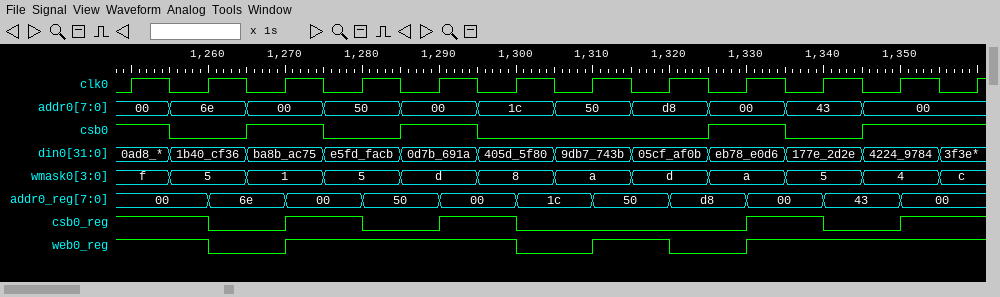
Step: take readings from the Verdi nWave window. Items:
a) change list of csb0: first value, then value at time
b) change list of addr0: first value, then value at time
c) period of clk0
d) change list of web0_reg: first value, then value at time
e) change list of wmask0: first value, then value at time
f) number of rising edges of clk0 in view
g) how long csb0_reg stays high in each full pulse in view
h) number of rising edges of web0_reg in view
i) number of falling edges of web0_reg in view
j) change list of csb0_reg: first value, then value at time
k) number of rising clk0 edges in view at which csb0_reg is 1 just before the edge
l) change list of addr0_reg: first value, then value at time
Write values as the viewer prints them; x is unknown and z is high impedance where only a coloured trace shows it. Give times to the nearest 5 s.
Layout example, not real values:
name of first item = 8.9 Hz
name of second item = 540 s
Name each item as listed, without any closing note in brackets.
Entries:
change list of csb0: first value, then value at time = 1, 0 at 1255 s, 1 at 1265 s, 0 at 1275 s, 1 at 1285 s, 0 at 1295 s, 1 at 1325 s, 0 at 1335 s, 1 at 1345 s
change list of addr0: first value, then value at time = 00, 6e at 1255 s, 00 at 1265 s, 50 at 1275 s, 00 at 1285 s, 1c at 1295 s, 50 at 1305 s, d8 at 1315 s, 00 at 1325 s, 43 at 1335 s, 00 at 1345 s
period of clk0 = 10 s
change list of web0_reg: first value, then value at time = 1, 0 at 1260 s, 1 at 1270 s, 0 at 1300 s, 1 at 1310 s, 0 at 1320 s, 1 at 1330 s
change list of wmask0: first value, then value at time = f, 5 at 1255 s, 1 at 1265 s, 5 at 1275 s, d at 1285 s, 8 at 1295 s, a at 1305 s, d at 1315 s, a at 1325 s, 5 at 1335 s, 4 at 1345 s, c at 1355 s
number of rising edges of clk0 in view = 12
how long csb0_reg stays high in each full pulse in view = 10 s, 10 s, 10 s
number of rising edges of web0_reg in view = 3
number of falling edges of web0_reg in view = 3
change list of csb0_reg: first value, then value at time = 1, 0 at 1260 s, 1 at 1270 s, 0 at 1280 s, 1 at 1290 s, 0 at 1300 s, 1 at 1330 s, 0 at 1340 s, 1 at 1350 s
number of rising clk0 edges in view at which csb0_reg is 1 just before the edge = 6
change list of addr0_reg: first value, then value at time = 00, 6e at 1260 s, 00 at 1270 s, 50 at 1280 s, 00 at 1290 s, 1c at 1300 s, 50 at 1310 s, d8 at 1320 s, 00 at 1330 s, 43 at 1340 s, 00 at 1350 s
